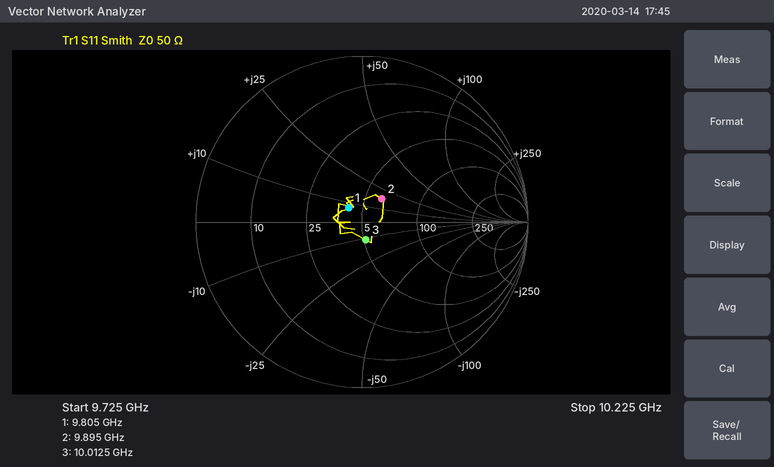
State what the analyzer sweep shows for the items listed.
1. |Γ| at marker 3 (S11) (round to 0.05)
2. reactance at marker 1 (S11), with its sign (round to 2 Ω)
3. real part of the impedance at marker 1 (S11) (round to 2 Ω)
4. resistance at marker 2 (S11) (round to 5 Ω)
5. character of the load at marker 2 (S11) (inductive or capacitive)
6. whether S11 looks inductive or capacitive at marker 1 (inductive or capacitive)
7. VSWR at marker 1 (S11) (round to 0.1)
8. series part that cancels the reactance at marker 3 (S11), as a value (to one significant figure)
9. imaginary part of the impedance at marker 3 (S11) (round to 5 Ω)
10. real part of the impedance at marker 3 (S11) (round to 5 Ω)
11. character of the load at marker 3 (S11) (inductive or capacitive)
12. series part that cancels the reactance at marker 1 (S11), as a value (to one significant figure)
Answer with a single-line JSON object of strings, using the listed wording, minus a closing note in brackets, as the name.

{"|Γ| at marker 3 (S11)": "0.10", "reactance at marker 1 (S11), with its sign": "+8 Ω", "real part of the impedance at marker 1 (S11)": "42 Ω", "resistance at marker 2 (S11)": "60 Ω", "character of the load at marker 2 (S11)": "inductive", "whether S11 looks inductive or capacitive at marker 1": "inductive", "VSWR at marker 1 (S11)": "1.3", "series part that cancels the reactance at marker 3 (S11), as a value": "200 pH", "imaginary part of the impedance at marker 3 (S11)": "-10 Ω", "real part of the impedance at marker 3 (S11)": "50 Ω", "character of the load at marker 3 (S11)": "capacitive", "series part that cancels the reactance at marker 1 (S11), as a value": "2 pF"}
